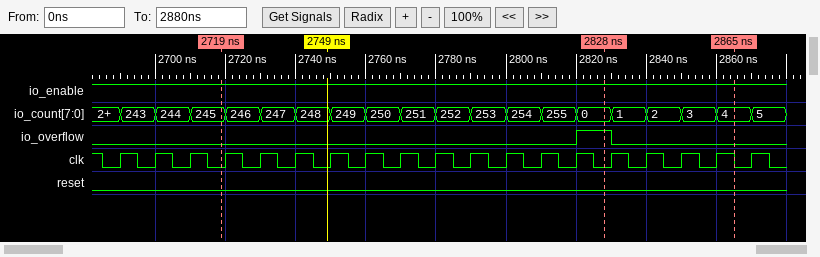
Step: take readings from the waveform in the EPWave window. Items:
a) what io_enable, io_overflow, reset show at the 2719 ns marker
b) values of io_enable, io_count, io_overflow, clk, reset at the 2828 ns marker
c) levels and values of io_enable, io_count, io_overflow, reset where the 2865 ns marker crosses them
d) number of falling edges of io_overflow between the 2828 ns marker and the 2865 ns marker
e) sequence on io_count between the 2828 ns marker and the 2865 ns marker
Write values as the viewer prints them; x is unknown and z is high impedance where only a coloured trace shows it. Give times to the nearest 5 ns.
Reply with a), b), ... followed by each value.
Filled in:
a) io_enable=1, io_overflow=0, reset=0
b) io_enable=1, io_count=0, io_overflow=1, clk=0, reset=0
c) io_enable=1, io_count=4, io_overflow=0, reset=0
d) 1
e) 0, 1, 2, 3, 4
